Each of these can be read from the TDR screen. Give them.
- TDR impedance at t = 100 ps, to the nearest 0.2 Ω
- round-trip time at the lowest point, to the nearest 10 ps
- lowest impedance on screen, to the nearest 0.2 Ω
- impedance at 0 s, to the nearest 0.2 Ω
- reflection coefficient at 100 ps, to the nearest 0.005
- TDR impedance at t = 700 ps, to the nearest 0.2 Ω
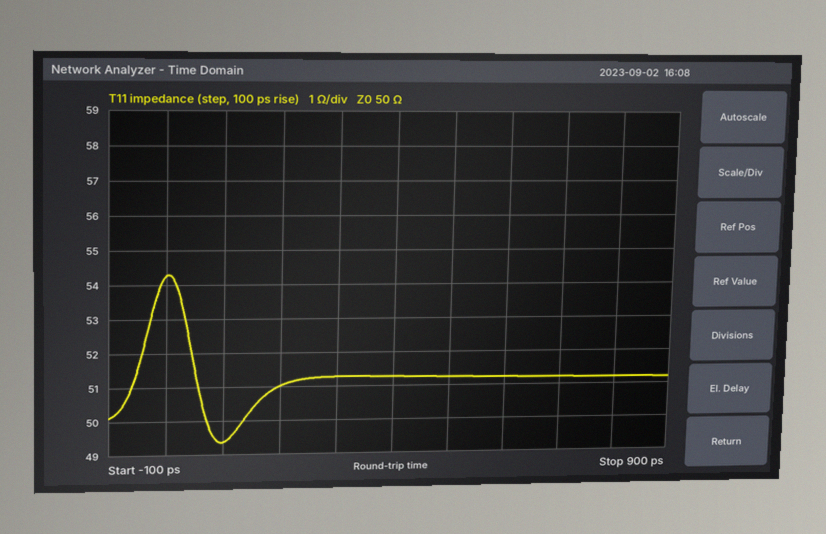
49.4 Ω
100 ps
49.4 Ω
54.2 Ω
-0.005
51.2 Ω
